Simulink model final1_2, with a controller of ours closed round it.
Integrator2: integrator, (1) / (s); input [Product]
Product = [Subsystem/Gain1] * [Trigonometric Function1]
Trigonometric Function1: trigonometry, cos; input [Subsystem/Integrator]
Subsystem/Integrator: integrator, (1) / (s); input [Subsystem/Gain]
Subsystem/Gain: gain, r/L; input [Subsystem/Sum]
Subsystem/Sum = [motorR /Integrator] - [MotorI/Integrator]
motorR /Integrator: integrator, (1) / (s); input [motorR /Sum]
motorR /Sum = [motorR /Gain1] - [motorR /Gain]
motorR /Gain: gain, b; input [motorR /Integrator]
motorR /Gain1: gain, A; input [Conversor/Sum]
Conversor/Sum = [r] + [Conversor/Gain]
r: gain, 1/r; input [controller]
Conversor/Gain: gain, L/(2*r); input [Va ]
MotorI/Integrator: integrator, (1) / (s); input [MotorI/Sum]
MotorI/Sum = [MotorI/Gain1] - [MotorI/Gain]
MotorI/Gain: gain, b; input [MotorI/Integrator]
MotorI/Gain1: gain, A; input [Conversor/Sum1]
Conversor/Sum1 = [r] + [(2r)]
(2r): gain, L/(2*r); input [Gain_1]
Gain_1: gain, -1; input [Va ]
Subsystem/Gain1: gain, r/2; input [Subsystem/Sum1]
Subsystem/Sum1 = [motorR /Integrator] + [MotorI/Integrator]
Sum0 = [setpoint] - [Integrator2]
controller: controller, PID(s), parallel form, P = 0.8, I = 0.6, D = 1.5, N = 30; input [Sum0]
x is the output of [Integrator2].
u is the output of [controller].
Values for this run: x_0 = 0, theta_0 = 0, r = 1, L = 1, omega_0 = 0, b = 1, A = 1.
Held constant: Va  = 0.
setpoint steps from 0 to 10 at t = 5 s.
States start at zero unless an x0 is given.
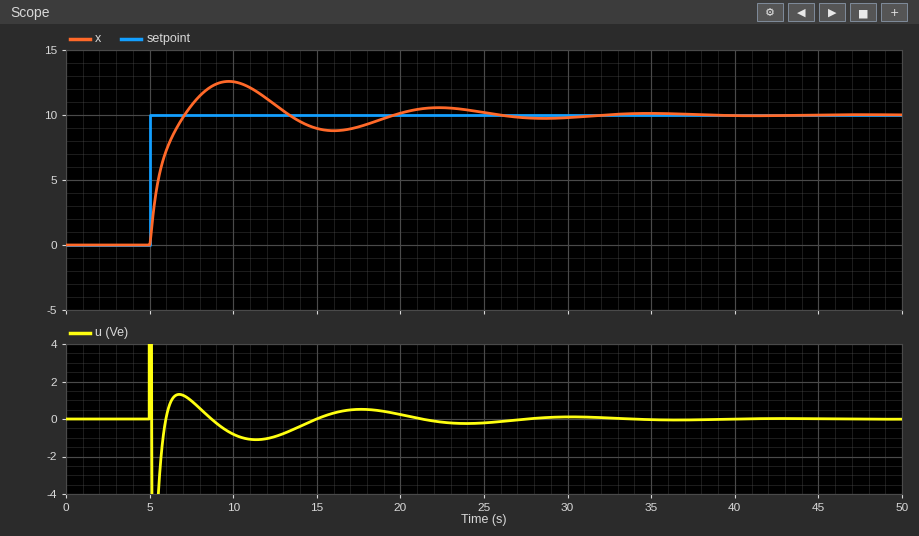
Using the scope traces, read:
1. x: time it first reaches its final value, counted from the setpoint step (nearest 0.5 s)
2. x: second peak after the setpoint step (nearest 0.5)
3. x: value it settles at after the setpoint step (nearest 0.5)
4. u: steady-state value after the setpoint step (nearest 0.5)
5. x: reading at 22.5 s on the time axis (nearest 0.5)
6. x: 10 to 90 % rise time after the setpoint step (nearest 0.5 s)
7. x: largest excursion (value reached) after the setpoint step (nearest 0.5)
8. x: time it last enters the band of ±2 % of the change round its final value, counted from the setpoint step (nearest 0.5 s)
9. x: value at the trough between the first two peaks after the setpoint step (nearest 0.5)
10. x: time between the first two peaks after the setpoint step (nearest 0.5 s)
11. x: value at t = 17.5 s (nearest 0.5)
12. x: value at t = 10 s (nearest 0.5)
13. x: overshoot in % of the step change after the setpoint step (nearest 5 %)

2.0 s
10.5
10.0
0.0
10.5
1.5 s
12.5
25.0 s
9.0
12.5 s
9.0
12.5
25 %
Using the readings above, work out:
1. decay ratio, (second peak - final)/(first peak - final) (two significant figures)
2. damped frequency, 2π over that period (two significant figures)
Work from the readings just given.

0.20
0.50 rad/s
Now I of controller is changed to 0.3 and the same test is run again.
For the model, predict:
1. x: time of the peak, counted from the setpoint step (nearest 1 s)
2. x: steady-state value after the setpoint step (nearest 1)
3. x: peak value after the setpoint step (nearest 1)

6 s
10
12
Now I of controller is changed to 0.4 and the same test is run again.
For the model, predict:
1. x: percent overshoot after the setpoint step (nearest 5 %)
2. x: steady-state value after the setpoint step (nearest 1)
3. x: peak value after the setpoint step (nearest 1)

20 %
10
12
